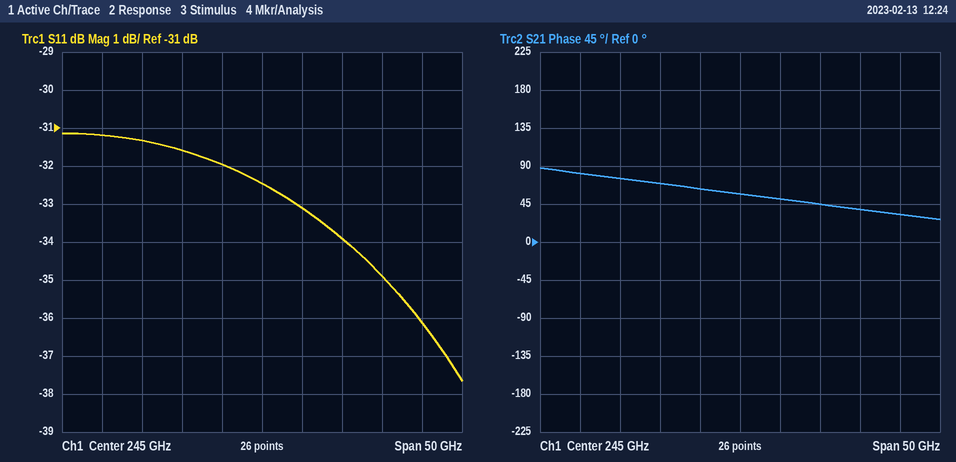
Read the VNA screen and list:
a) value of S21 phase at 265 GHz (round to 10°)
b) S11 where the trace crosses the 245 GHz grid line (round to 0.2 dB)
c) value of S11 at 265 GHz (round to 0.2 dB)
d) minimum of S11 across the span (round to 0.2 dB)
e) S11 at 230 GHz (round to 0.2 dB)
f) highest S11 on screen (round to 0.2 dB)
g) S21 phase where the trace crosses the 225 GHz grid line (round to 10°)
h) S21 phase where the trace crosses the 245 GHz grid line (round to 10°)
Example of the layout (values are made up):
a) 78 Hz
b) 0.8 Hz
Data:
a) 30°
b) -32.4 dB
c) -36.2 dB
d) -37.6 dB
e) -31.4 dB
f) -31.2 dB
g) 80°
h) 60°
